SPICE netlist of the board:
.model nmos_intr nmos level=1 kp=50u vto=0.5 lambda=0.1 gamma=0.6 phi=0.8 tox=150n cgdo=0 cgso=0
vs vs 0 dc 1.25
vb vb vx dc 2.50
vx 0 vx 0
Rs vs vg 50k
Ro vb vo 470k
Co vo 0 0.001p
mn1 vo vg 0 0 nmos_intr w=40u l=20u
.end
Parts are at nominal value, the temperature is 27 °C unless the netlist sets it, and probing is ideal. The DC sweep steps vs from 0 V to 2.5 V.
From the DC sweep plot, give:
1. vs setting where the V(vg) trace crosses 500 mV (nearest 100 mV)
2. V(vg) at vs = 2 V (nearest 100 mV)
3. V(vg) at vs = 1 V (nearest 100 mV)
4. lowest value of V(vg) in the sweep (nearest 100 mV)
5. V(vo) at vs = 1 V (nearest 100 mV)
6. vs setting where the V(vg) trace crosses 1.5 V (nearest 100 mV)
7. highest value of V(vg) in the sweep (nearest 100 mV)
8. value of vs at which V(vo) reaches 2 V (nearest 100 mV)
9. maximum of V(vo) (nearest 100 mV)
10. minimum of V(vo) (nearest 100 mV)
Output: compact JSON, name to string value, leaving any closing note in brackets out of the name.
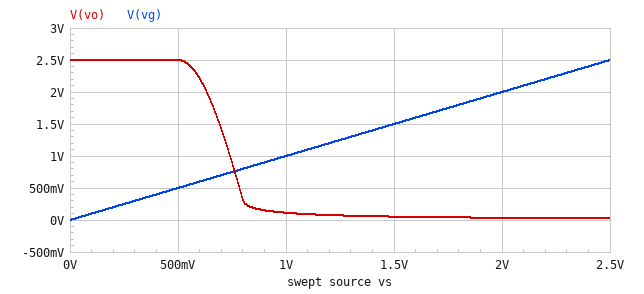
{"vs setting where the V(vg) trace crosses 500 mV": "500 mV", "V(vg) at vs = 2 V": "2.0 V", "V(vg) at vs = 1 V": "1.0 V", "lowest value of V(vg) in the sweep": "0 V", "V(vo) at vs = 1 V": "100 mV", "vs setting where the V(vg) trace crosses 1.5 V": "1.5 V", "highest value of V(vg) in the sweep": "2.5 V", "value of vs at which V(vo) reaches 2 V": "600 mV", "maximum of V(vo)": "2.5 V", "minimum of V(vo)": "0 V"}
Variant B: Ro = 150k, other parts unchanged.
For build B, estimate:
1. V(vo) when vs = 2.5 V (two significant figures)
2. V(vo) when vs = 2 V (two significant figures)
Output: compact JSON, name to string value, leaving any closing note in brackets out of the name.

{"V(vo) when vs = 2.5 V": "82 mV", "V(vo) when vs = 2 V": "110 mV"}
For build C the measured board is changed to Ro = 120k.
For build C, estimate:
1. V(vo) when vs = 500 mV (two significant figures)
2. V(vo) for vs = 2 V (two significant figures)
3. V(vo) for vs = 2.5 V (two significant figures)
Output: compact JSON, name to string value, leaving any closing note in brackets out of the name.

{"V(vo) when vs = 500 mV": "2.5 V", "V(vo) for vs = 2 V": "140 mV", "V(vo) for vs = 2.5 V": "100 mV"}
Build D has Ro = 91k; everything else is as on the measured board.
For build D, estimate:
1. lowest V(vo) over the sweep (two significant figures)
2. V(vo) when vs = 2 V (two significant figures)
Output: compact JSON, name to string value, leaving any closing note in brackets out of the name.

{"lowest V(vo) over the sweep": "130 mV", "V(vo) when vs = 2 V": "180 mV"}
